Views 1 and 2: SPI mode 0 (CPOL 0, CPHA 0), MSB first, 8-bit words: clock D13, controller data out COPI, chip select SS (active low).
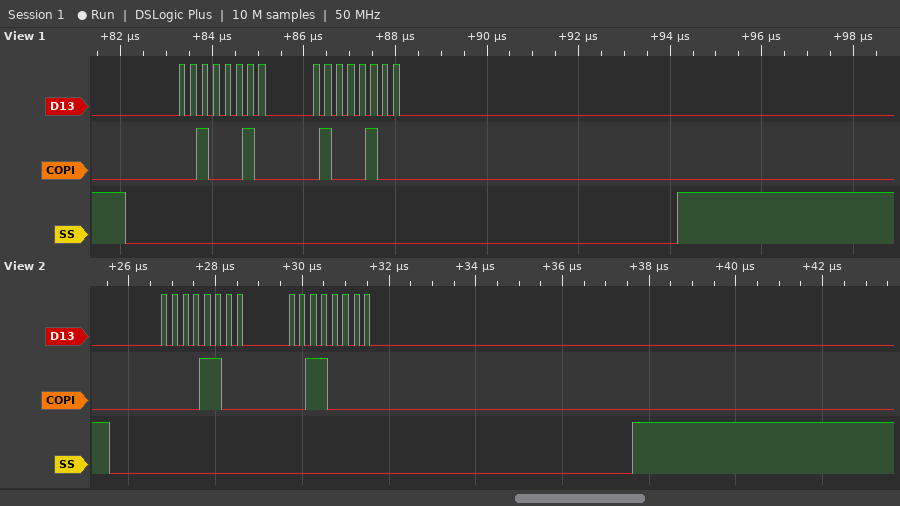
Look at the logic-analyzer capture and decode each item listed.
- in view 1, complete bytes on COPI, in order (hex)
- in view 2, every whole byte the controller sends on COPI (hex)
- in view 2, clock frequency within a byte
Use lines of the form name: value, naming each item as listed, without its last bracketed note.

in view 1, complete bytes on COPI, in order: 22 44
in view 2, every whole byte the controller sends on COPI: 0C 30
in view 2, clock frequency within a byte: 4 MHz
